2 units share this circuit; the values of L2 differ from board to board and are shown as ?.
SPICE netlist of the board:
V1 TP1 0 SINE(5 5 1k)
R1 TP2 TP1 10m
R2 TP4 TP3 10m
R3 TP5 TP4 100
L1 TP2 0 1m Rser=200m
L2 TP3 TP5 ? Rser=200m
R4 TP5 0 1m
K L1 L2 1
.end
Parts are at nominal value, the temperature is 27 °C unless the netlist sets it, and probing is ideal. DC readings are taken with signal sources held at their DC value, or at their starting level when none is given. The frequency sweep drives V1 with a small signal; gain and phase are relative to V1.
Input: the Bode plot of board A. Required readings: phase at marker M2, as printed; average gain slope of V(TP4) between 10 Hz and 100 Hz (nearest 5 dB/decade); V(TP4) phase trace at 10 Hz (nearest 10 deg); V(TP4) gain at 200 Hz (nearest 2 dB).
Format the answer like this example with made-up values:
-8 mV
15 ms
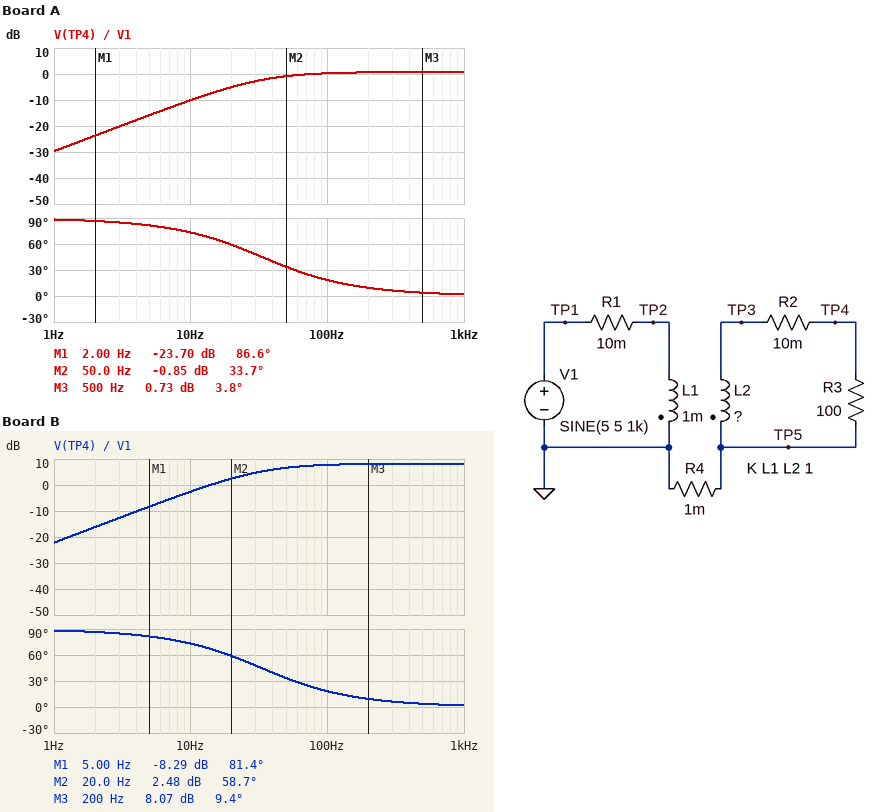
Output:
33.7 deg
10 dB/decade
70 deg
0 dB
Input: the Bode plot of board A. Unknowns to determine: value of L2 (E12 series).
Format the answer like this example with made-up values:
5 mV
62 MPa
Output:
1.2 mH
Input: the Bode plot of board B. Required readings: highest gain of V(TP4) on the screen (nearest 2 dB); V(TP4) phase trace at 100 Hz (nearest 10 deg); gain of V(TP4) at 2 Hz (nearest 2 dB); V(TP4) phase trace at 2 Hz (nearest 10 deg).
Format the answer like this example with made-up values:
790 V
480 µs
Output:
8 dB
20 deg
-16 dB
90 deg
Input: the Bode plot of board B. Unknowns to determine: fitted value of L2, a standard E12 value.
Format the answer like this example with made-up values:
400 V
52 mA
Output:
6.8 mH
